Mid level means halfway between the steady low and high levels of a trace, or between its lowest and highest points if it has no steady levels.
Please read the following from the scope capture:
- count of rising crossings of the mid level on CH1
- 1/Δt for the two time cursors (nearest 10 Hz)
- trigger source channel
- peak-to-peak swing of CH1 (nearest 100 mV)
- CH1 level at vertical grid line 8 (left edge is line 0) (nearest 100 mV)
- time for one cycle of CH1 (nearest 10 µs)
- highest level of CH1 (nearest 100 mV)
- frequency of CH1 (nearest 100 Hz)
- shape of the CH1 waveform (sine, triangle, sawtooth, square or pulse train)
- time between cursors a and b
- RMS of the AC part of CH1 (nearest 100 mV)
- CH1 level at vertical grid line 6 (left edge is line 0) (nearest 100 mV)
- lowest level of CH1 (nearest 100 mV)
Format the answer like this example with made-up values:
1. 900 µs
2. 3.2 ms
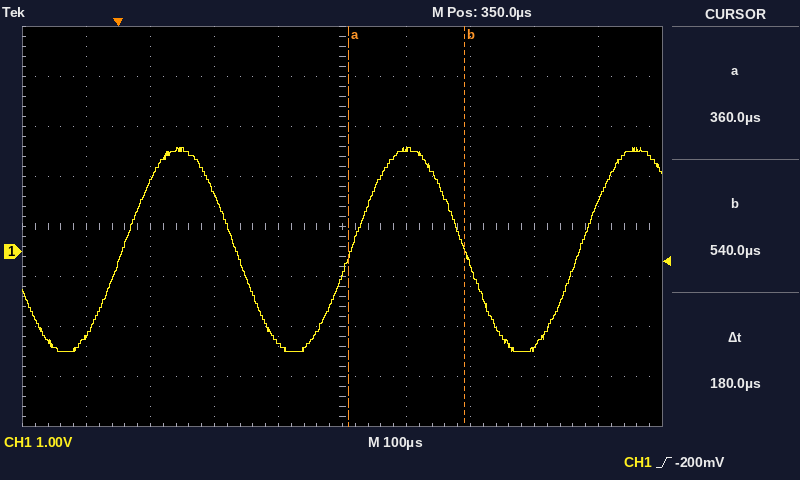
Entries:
1. 3
2. 5.56 kHz
3. CH1
4. 4.1 V
5. -1.9 V
6. 360 µs
7. 2.1 V
8. 2.8 kHz
9. sine
10. 180 µs
11. 1.4 V
12. 2.0 V
13. -2.0 V
